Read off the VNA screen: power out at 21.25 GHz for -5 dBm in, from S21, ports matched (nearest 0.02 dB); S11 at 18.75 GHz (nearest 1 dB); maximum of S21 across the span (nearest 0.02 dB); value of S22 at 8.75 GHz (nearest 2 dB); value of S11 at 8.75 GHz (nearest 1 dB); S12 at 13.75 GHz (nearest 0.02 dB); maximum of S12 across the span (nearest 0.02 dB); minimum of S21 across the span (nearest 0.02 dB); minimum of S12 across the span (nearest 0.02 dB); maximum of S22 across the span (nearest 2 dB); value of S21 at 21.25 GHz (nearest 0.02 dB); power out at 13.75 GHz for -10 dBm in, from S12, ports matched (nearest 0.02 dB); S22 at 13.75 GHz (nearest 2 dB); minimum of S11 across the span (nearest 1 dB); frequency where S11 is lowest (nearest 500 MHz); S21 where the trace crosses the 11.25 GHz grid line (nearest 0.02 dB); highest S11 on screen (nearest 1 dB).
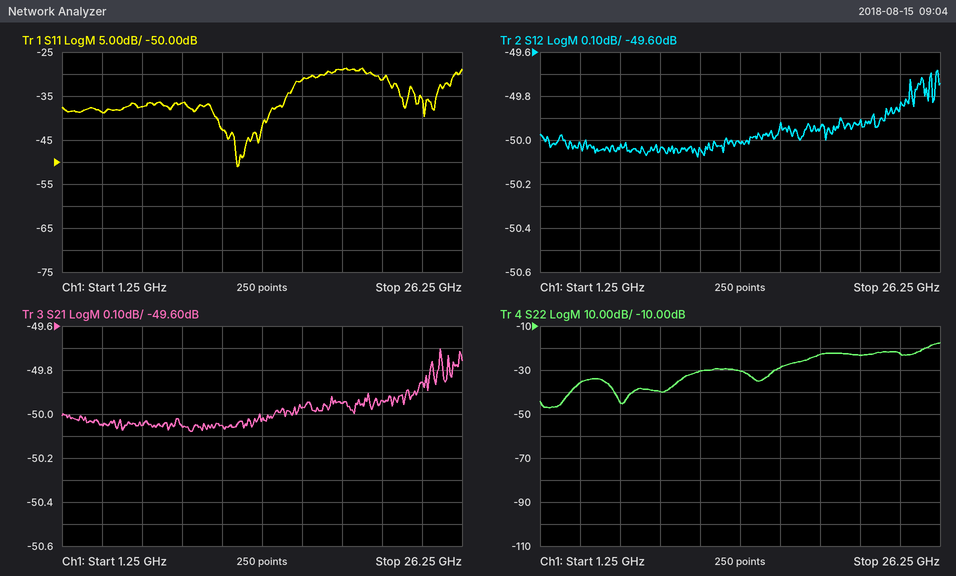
-54.94 dBm
-29 dB
-49.70 dB
-40 dB
-37 dB
-50.02 dB
-49.68 dB
-50.08 dB
-50.08 dB
-18 dB
-49.94 dB
-60.02 dBm
-30 dB
-51 dB
12.0 GHz
-50.06 dB
-29 dB
